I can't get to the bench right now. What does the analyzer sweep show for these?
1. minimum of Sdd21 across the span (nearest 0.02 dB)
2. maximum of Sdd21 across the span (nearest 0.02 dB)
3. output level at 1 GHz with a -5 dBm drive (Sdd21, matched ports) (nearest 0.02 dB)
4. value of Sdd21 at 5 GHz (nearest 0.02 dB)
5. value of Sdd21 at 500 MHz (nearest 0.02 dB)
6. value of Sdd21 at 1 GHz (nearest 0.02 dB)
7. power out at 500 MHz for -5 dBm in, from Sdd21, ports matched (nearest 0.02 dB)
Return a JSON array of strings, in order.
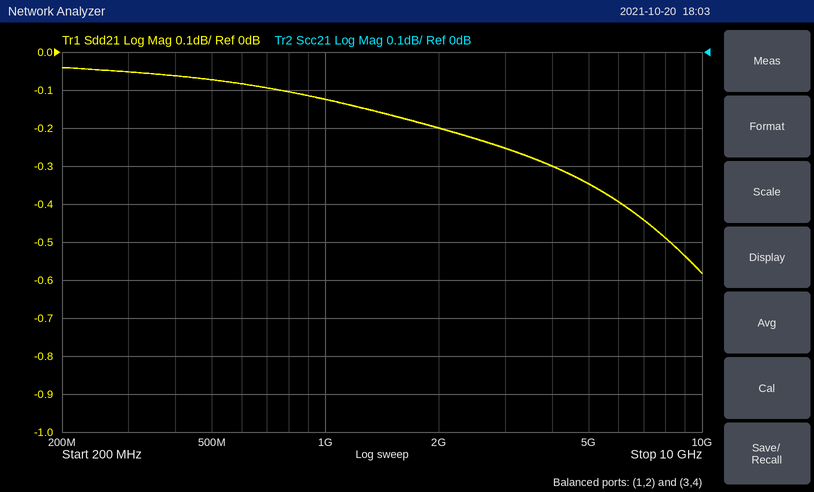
["-0.58 dB", "-0.04 dB", "-5.12 dBm", "-0.34 dB", "-0.08 dB", "-0.12 dB", "-5.08 dBm"]
